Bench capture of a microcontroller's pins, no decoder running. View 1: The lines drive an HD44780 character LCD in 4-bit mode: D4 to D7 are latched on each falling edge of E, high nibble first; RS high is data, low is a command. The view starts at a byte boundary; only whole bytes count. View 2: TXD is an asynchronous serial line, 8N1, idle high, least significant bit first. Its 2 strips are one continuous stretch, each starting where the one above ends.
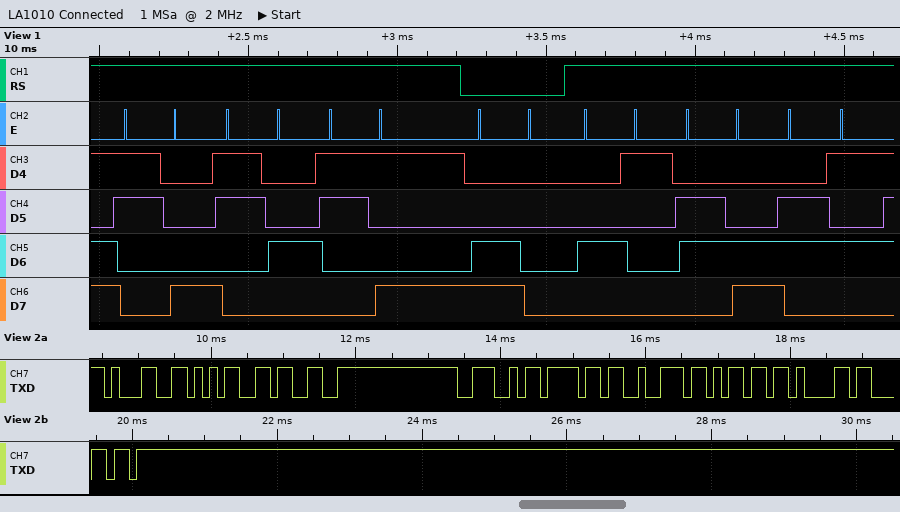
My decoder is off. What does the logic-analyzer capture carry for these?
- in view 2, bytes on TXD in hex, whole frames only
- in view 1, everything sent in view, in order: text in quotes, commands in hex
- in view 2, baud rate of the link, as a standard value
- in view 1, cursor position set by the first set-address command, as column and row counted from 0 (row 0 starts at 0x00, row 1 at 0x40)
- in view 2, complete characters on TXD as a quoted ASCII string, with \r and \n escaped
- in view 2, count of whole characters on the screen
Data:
31 35 33 4E 6F 72 6D 61 6C
"849" 0xC0 "Ale"
9600 baud
column 0, row 1
"153Normal"
9
